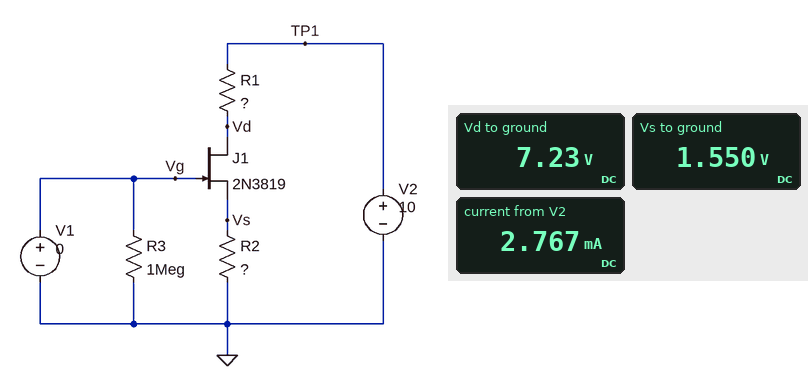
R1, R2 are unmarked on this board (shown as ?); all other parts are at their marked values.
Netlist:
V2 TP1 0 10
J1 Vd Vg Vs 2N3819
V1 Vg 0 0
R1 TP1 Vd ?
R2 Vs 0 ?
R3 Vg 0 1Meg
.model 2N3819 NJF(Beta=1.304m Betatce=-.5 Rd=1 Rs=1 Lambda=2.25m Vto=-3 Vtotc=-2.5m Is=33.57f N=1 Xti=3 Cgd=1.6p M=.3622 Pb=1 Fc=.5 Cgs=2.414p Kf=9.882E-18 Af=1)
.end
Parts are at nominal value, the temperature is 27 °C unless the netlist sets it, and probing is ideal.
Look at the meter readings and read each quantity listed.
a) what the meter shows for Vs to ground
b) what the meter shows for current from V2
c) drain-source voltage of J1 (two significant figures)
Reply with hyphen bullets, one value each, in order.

- 1.550 V
- 2.767 mA
- 5.7 V
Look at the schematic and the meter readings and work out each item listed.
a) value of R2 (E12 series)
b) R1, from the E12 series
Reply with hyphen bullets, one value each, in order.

- 560 Ω
- 1 kΩ
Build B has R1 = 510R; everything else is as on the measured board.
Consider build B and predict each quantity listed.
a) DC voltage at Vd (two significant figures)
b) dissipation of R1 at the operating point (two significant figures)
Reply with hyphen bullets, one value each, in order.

- 8.6 V
- 3.9 mW
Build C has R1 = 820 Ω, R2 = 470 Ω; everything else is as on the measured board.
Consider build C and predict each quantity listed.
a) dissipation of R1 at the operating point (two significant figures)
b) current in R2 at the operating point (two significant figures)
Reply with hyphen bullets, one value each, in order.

- 7.9 mW
- 3.1 mA
